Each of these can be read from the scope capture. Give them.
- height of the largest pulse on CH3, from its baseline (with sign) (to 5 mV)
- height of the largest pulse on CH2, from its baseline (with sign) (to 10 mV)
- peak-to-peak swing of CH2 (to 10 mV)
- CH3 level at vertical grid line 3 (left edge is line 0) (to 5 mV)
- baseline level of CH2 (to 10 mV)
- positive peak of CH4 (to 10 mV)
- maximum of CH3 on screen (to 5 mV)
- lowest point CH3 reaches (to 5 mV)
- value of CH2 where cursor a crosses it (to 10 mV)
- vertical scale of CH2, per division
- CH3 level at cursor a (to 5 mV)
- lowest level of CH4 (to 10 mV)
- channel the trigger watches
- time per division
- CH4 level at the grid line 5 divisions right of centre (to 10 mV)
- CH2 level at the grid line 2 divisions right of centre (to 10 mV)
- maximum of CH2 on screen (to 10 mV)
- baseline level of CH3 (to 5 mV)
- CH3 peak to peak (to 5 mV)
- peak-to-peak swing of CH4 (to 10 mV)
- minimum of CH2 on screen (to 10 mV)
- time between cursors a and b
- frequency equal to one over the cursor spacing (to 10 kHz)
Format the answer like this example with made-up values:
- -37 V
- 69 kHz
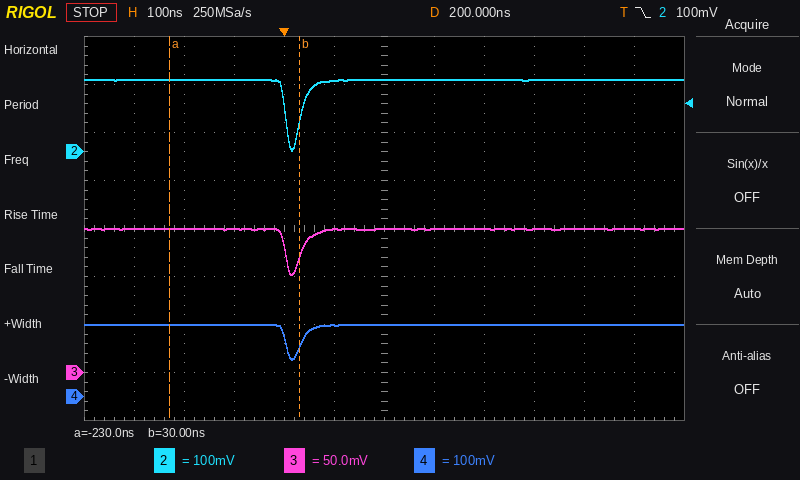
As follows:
- -50 mV
- -150 mV
- 150 mV
- 150 mV
- 150 mV
- 150 mV
- 150 mV
- 100 mV
- 150 mV
- 100 mV
- 150 mV
- 80 mV
- CH2
- 100 ns
- 150 mV
- 150 mV
- 150 mV
- 150 mV
- 50 mV
- 70 mV
- 0 mV
- 260 ns
- 3.85 MHz
